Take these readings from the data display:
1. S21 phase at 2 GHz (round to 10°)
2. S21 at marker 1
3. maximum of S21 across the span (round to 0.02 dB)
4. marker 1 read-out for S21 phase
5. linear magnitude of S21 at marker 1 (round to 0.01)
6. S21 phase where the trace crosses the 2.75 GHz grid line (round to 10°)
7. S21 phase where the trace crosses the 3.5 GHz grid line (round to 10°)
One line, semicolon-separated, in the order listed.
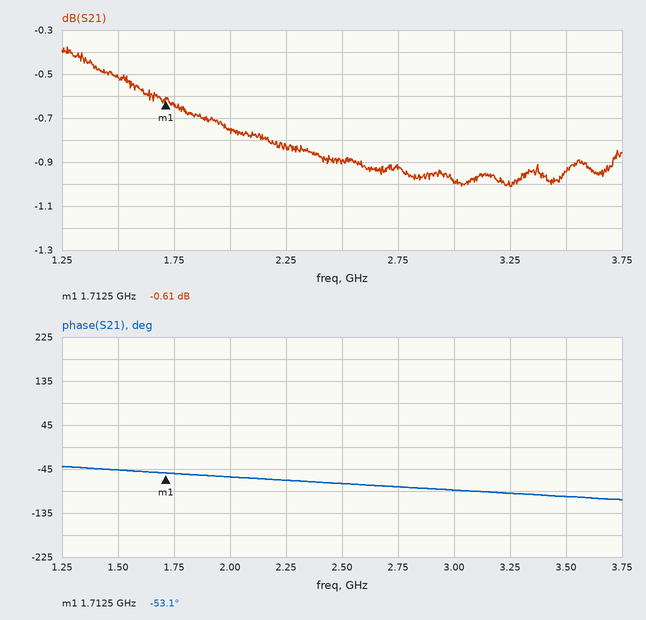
-60°; -0.61 dB; -0.38 dB; -53.1°; 0.93; -80°; -100°
